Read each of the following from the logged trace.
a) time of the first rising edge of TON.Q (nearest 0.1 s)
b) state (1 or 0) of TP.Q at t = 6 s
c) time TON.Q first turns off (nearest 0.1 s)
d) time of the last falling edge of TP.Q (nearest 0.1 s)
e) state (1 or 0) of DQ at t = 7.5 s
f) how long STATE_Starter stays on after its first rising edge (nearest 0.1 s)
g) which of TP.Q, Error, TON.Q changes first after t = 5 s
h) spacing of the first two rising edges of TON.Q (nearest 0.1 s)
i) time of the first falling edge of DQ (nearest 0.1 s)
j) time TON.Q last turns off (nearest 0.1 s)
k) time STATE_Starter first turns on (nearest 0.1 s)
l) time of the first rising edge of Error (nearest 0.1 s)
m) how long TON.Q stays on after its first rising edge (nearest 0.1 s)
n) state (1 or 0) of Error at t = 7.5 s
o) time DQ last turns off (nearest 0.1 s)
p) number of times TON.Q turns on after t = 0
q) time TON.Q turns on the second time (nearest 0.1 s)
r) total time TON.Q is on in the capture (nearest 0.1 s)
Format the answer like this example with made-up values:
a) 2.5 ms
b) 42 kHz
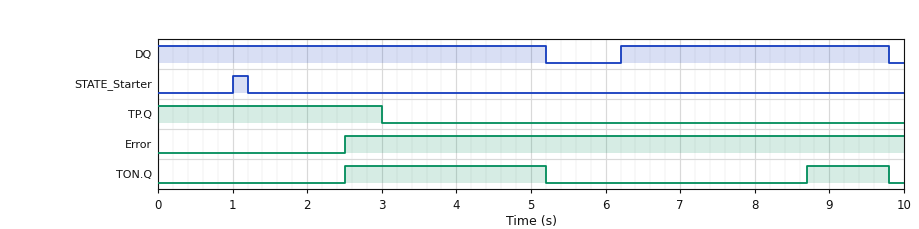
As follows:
a) 2.5 s
b) 0
c) 5.2 s
d) 3.0 s
e) 1
f) 0.2 s
g) TON.Q
h) 6.2 s
i) 5.2 s
j) 9.8 s
k) 1.0 s
l) 2.5 s
m) 2.7 s
n) 1
o) 9.8 s
p) 2
q) 8.7 s
r) 3.8 s
